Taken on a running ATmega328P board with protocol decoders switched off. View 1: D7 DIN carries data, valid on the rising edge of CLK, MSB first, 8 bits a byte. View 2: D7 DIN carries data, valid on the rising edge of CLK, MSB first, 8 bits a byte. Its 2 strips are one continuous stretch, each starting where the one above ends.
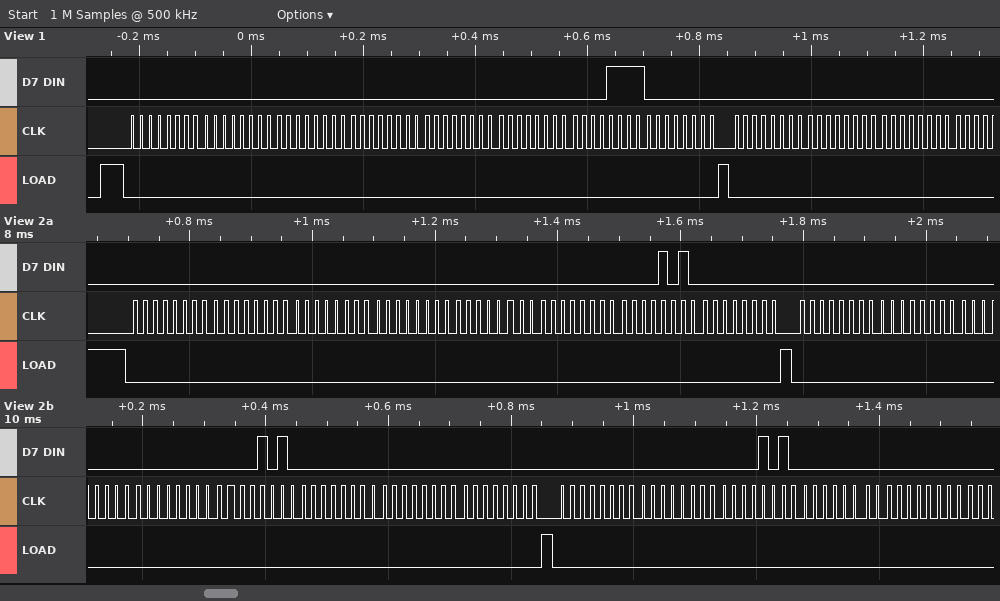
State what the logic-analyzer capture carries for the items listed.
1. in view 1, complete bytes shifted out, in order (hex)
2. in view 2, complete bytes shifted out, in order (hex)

00 00 00 00 00 00 0F 00 00 00 00
0x00 0x00 0x00 0x00 0x00 0x00 0x0A 0x00 0x00 0x00 0x00 0x00 0x0A 0x00 0x00 0x00 0x00 0x00 0x0A 0x00 0x00
